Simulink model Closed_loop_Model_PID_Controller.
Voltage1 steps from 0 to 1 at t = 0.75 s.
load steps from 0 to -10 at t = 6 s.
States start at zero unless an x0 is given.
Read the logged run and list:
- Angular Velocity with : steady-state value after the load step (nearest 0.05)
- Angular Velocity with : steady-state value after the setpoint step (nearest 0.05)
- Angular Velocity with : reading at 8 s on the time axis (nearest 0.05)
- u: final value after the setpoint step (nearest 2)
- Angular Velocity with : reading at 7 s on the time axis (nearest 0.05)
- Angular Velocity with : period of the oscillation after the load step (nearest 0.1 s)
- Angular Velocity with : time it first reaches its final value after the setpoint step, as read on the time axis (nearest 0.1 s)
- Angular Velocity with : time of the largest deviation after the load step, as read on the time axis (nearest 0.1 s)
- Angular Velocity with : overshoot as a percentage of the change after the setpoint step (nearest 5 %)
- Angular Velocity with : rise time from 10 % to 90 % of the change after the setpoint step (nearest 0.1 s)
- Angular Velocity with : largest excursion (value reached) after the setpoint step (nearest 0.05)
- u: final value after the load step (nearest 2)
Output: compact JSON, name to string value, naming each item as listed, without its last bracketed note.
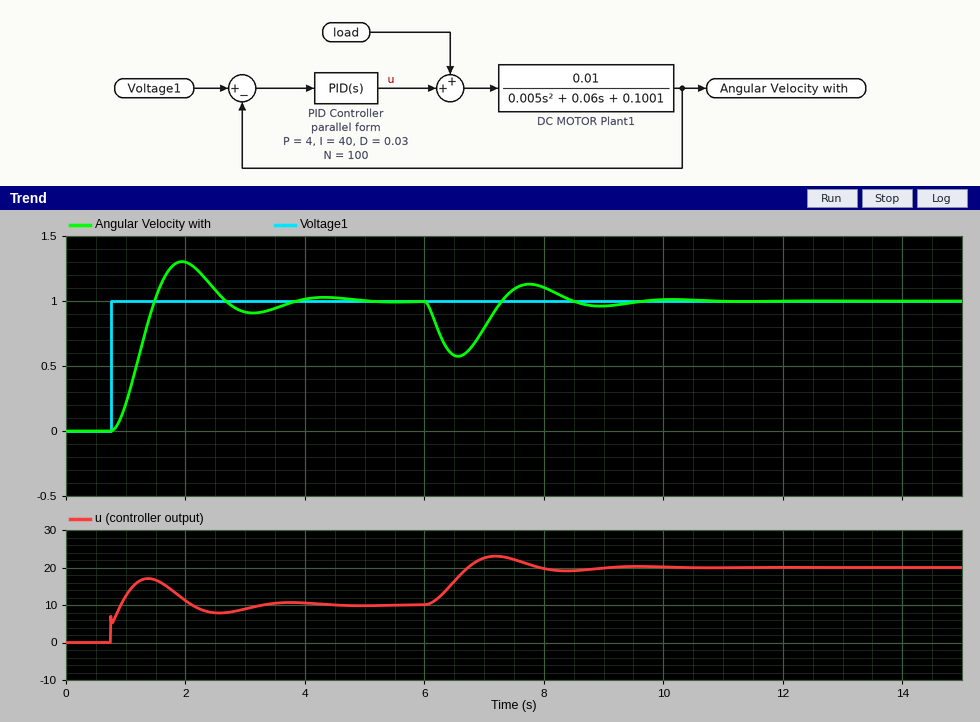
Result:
{"Angular Velocity with : steady-state value after the load step": "1.00", "Angular Velocity with : steady-state value after the setpoint step": "1.00", "Angular Velocity with : reading at 8 s on the time axis": "1.10", "u: final value after the setpoint step": "10", "Angular Velocity with : reading at 7 s on the time axis": "0.80", "Angular Velocity with : period of the oscillation after the load step": "2.4 s", "Angular Velocity with : time it first reaches its final value after the setpoint step, as read on the time axis": "1.5 s", "Angular Velocity with : time of the largest deviation after the load step, as read on the time axis": "6.6 s", "Angular Velocity with : overshoot as a percentage of the change after the setpoint step": "30 %", "Angular Velocity with : rise time from 10 % to 90 % of the change after the setpoint step": "0.5 s", "Angular Velocity with : largest excursion (value reached) after the setpoint step": "1.30", "u: final value after the load step": "20"}
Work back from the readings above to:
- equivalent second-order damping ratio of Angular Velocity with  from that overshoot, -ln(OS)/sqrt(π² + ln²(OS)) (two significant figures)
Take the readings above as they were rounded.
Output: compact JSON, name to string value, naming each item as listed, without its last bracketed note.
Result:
{"equivalent second-order damping ratio of Angular Velocity with  from that overshoot, -ln(OS)/sqrt(π² + ln²(OS))": "0.36"}
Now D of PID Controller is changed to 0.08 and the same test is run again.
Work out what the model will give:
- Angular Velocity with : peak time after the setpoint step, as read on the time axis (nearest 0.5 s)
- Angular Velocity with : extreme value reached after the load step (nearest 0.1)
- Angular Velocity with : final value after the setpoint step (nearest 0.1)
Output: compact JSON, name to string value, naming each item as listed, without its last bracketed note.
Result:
{"Angular Velocity with : peak time after the setpoint step, as read on the time axis": "2.0 s", "Angular Velocity with : extreme value reached after the load step": "0.6", "Angular Velocity with : final value after the setpoint step": "1.0"}
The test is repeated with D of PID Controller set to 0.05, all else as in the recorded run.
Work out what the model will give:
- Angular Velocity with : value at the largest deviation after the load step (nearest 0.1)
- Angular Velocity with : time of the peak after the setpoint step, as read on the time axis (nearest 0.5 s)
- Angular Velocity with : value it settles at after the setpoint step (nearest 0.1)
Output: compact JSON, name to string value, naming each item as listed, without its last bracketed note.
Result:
{"Angular Velocity with : value at the largest deviation after the load step": "0.6", "Angular Velocity with : time of the peak after the setpoint step, as read on the time axis": "2.0 s", "Angular Velocity with : value it settles at after the setpoint step": "1.0"}
